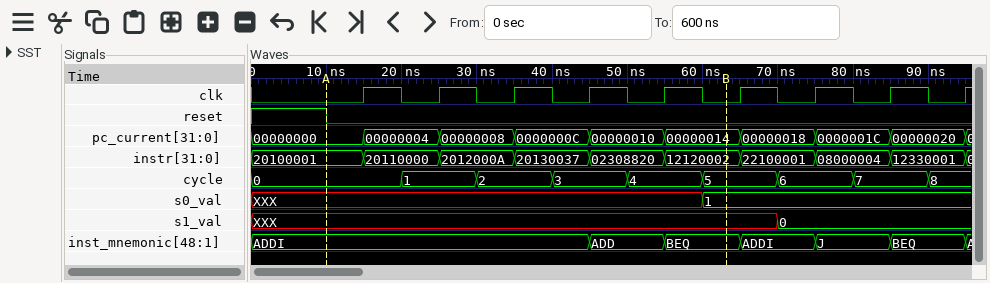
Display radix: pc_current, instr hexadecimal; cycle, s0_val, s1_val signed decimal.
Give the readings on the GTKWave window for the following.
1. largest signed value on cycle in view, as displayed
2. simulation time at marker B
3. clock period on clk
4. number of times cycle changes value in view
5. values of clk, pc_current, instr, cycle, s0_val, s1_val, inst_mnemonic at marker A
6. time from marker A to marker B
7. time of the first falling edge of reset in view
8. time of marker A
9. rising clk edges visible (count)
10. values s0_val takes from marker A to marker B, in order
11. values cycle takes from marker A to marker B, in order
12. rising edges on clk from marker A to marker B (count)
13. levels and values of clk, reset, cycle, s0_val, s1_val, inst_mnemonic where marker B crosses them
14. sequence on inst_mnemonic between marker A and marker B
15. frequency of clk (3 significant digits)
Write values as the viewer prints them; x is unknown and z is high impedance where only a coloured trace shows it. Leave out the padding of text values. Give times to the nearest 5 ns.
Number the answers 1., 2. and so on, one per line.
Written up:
1. 8
2. 65 ns
3. 10 ns
4. 8
5. clk=0, pc_current=00000000, instr=20100001, cycle=0, s0_val=XXX, s1_val=XXX, inst_mnemonic=ADDI
6. 55 ns
7. 10 ns
8. 10 ns
9. 9
10. XXX, 1
11. 0, 1, 2, 3, 4, 5
12. 5
13. clk=0, reset=0, cycle=5, s0_val=1, s1_val=XXX, inst_mnemonic=BEQ
14. ADDI, ADD, BEQ
15. 100 MHz
